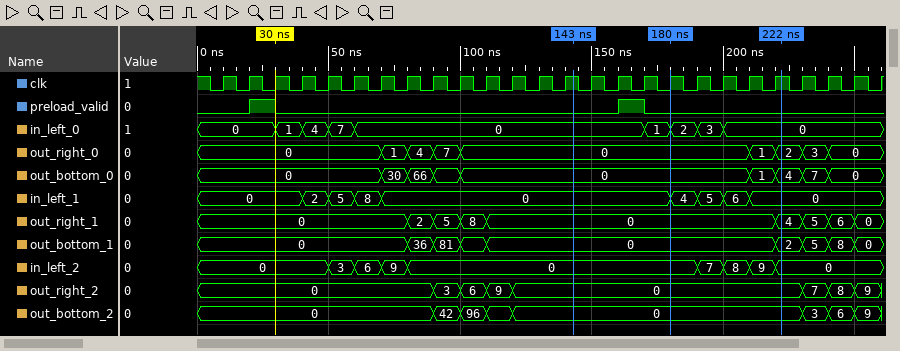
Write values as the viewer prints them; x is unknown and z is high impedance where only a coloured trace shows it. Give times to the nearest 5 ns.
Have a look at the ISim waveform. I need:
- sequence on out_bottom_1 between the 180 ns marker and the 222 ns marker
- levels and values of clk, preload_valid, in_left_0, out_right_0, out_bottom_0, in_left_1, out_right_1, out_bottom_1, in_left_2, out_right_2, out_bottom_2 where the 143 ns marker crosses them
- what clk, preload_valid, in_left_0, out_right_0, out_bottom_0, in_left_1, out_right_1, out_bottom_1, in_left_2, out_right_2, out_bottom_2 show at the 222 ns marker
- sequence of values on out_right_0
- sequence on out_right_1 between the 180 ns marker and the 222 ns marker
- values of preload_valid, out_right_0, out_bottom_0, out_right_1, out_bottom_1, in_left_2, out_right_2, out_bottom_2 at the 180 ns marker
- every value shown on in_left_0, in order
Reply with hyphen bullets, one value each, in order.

- 0, 2
- clk=1, preload_valid=0, in_left_0=0, out_right_0=0, out_bottom_0=0, in_left_1=0, out_right_1=0, out_bottom_1=0, in_left_2=0, out_right_2=0, out_bottom_2=0
- clk=1, preload_valid=0, in_left_0=0, out_right_0=2, out_bottom_0=4, in_left_1=0, out_right_1=4, out_bottom_1=2, in_left_2=0, out_right_2=0, out_bottom_2=0
- 0, 1, 4, 7, 0, 1, 2, 3, 0
- 0, 4
- preload_valid=0, out_right_0=0, out_bottom_0=0, out_right_1=0, out_bottom_1=0, in_left_2=0, out_right_2=0, out_bottom_2=0
- 0, 1, 4, 7, 0, 1, 2, 3, 0
